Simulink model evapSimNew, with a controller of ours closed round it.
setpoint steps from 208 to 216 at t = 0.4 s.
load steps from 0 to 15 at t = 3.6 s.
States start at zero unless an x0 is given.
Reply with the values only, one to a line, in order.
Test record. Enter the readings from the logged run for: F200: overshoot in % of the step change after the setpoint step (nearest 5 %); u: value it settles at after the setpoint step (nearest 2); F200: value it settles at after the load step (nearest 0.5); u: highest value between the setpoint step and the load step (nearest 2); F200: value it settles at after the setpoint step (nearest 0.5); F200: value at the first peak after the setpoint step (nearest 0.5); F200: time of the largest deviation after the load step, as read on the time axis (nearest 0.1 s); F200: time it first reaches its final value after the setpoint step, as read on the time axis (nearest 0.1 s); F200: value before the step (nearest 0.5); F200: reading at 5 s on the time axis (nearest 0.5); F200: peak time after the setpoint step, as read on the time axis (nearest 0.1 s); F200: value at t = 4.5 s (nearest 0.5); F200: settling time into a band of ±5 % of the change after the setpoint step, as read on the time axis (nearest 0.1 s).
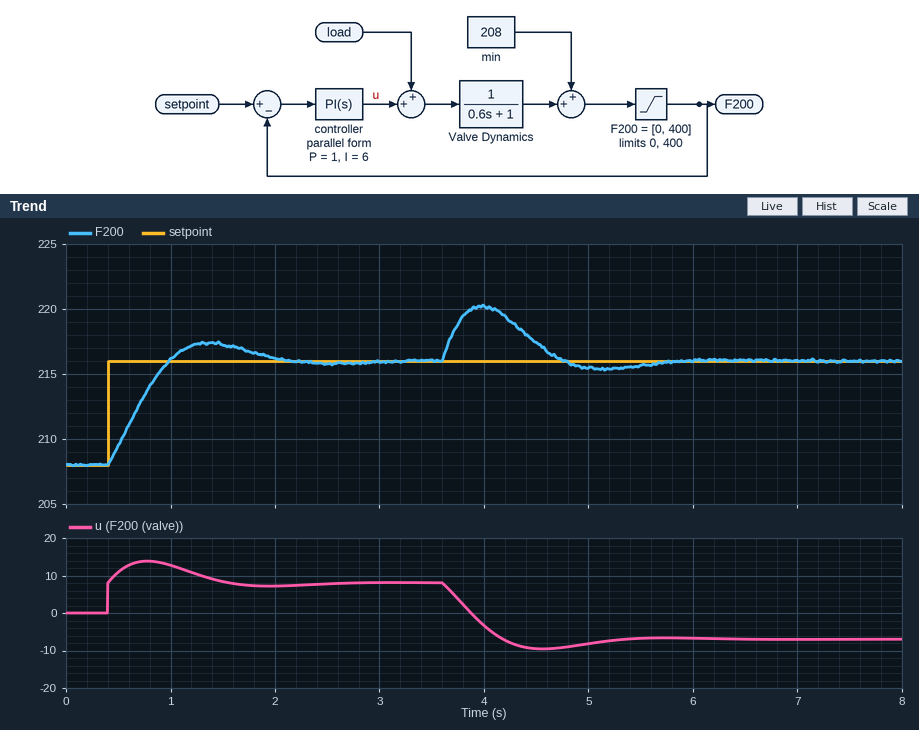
15 %
8
216.0
14
216.0
217.5
4.0 s
1.0 s
208.0
215.5
1.4 s
217.5
1.9 s
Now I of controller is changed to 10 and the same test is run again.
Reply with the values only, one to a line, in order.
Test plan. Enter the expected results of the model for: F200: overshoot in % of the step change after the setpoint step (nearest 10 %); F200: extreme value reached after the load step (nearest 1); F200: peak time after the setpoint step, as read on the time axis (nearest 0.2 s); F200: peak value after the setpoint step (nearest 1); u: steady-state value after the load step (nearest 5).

30 %
220
1.2 s
218
-5
